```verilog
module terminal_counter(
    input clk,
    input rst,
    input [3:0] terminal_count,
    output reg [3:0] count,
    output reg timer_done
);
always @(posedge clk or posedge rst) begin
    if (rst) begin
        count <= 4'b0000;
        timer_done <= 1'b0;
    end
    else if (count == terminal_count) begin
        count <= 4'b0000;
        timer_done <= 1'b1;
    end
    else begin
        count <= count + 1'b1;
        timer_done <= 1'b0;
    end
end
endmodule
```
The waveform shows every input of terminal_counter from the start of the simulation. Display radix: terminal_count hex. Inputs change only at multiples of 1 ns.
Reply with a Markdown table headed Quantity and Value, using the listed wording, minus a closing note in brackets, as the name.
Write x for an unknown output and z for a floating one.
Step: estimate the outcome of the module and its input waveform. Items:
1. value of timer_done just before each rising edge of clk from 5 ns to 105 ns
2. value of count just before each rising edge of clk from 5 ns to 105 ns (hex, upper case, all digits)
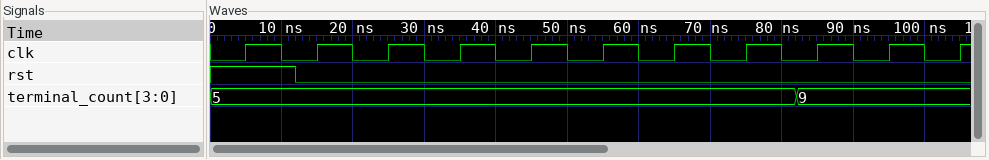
| Quantity | Value |
|---|---|
| value of timer_done just before each rising edge of clk from 5 ns to 105 ns | 0 0 0 0 0 0 0 1 0 0 0 |
| value of count just before each rising edge of clk from 5 ns to 105 ns | 0, 0, 1, 2, 3, 4, 5, 0, 1, 2, 3 |
